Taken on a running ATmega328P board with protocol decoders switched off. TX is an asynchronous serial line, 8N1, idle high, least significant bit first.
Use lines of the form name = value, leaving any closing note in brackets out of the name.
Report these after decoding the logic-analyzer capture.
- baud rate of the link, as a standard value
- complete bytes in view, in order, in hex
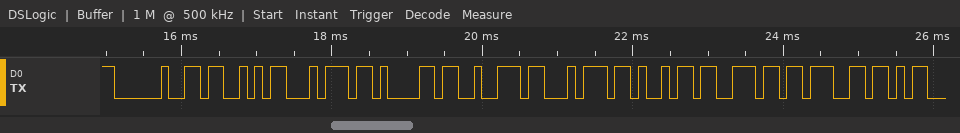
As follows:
baud rate of the link, as a standard value = 9600 baud
complete bytes in view, in order, in hex = 0x20 0x53 0x74 0x61 0x72 0x74 0x69 0x6E 0x67
